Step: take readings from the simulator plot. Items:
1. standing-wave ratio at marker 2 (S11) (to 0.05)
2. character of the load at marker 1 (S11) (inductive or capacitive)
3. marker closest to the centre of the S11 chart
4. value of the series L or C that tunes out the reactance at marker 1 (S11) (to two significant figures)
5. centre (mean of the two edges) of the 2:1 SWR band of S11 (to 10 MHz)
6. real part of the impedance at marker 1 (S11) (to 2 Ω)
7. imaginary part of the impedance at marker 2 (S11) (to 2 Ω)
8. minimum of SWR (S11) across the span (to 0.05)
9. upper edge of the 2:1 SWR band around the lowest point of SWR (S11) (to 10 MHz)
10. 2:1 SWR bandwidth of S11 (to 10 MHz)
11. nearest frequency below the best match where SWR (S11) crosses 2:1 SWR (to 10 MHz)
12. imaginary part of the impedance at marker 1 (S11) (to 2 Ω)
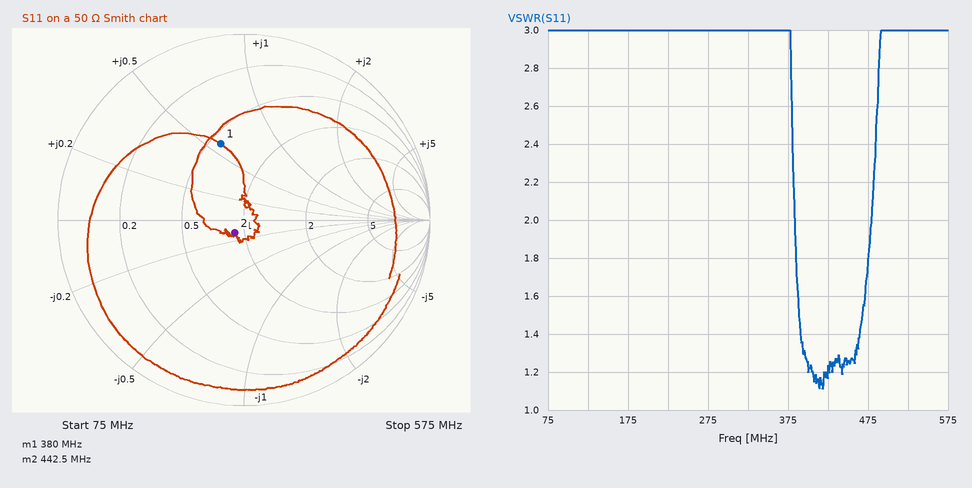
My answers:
1.20
inductive
marker 2
15 pF
430 MHz
28 Ω
-6 Ω
1.10
480 MHz
100 MHz
380 MHz
+28 Ω
